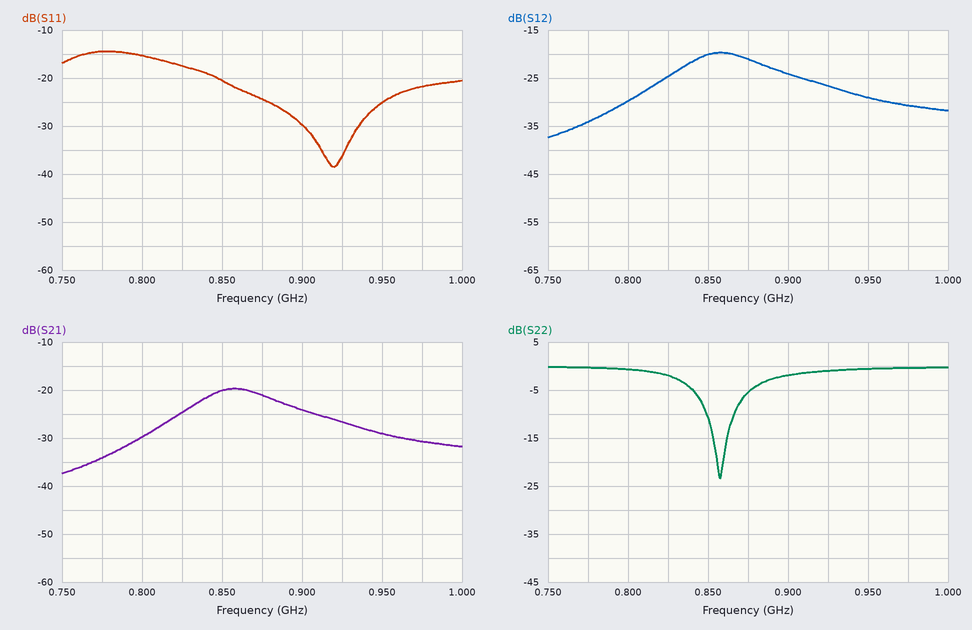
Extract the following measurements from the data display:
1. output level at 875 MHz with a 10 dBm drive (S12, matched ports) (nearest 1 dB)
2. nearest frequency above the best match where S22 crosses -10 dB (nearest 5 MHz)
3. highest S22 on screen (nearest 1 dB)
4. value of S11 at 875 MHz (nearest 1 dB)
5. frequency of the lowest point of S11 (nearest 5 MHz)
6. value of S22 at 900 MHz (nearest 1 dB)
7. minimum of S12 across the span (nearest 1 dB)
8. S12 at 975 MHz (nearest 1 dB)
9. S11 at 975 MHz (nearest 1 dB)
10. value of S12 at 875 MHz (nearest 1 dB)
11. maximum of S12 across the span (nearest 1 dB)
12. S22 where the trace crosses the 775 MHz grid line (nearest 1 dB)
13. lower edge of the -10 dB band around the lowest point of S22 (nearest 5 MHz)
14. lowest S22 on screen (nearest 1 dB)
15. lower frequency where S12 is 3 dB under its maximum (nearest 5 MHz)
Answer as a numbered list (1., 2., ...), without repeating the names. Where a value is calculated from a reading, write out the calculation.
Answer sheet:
1. 10 dBm + (-21 dB) = -11 dBm
2. 865 MHz
3. 0 dB
4. -24 dB
5. 920 MHz
6. -2 dB
7. -37 dB
8. -31 dB
9. -22 dB
10. -21 dB
11. -20 dB
12. 0 dB
13. 850 MHz
14. -23 dB
15. 835 MHz
